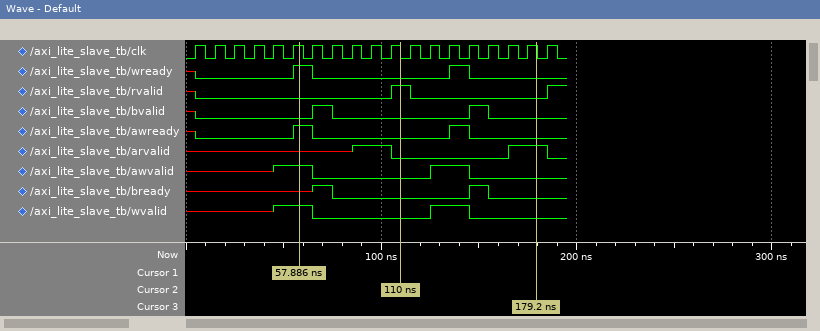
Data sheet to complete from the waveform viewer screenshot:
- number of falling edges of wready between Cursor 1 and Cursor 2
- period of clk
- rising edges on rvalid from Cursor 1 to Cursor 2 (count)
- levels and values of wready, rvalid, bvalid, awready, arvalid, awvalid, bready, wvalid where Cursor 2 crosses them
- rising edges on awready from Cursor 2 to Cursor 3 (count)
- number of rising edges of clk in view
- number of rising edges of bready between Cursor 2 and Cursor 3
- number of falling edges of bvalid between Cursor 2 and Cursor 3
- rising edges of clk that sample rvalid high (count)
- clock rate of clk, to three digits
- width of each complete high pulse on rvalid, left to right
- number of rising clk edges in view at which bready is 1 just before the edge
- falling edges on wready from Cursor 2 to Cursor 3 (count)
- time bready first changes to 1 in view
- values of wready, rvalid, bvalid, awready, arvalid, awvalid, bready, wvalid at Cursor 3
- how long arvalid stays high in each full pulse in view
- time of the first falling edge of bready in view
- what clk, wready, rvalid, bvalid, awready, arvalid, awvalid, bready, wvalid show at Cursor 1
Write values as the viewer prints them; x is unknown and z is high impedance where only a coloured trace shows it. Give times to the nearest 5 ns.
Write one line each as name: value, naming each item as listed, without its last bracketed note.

number of falling edges of wready between Cursor 1 and Cursor 2: 1
period of clk: 10 ns
rising edges on rvalid from Cursor 1 to Cursor 2: 1
levels and values of wready, rvalid, bvalid, awready, arvalid, awvalid, bready, wvalid where Cursor 2 crosses them: wready=0, rvalid=1, bvalid=0, awready=0, arvalid=0, awvalid=0, bready=0, wvalid=0
rising edges on awready from Cursor 2 to Cursor 3: 1
number of rising edges of clk in view: 19
number of rising edges of bready between Cursor 2 and Cursor 3: 1
number of falling edges of bvalid between Cursor 2 and Cursor 3: 1
rising edges of clk that sample rvalid high: 1
clock rate of clk, to three digits: 100 MHz
width of each complete high pulse on rvalid, left to right: 10 ns
number of rising clk edges in view at which bready is 1 just before the edge: 2
falling edges on wready from Cursor 2 to Cursor 3: 1
time bready first changes to 1 in view: 65 ns
values of wready, rvalid, bvalid, awready, arvalid, awvalid, bready, wvalid at Cursor 3: wready=0, rvalid=0, bvalid=0, awready=0, arvalid=1, awvalid=0, bready=0, wvalid=0
how long arvalid stays high in each full pulse in view: 20 ns
time of the first falling edge of bready in view: 75 ns
what clk, wready, rvalid, bvalid, awready, arvalid, awvalid, bready, wvalid show at Cursor 1: clk=1, wready=1, rvalid=0, bvalid=0, awready=1, arvalid=x, awvalid=1, bready=x, wvalid=1
